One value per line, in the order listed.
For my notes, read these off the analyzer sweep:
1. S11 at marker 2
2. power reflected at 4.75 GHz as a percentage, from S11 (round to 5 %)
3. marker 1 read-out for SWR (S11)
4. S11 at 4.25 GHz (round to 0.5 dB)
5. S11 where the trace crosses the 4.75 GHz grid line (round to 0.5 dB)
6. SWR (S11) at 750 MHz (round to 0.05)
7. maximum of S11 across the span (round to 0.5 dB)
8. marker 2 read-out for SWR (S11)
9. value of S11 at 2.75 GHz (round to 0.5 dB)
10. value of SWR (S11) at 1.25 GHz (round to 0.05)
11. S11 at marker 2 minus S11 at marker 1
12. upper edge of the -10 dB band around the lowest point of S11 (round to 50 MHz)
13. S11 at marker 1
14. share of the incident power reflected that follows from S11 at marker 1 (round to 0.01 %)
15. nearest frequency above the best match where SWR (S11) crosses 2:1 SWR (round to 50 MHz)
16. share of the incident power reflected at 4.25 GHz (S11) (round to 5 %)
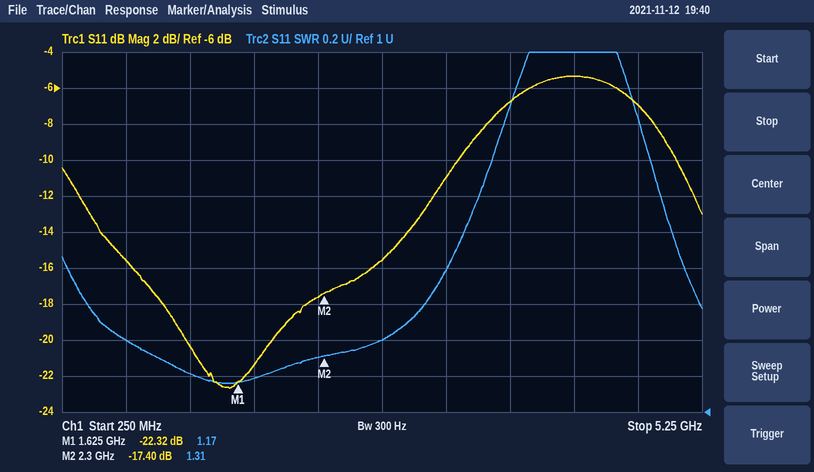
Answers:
-17.40 dB
20 %
1.17
-5.5 dB
-7.0 dB
1.40
-5.5 dB
1.31
-15.5 dB
1.20
4.92 dB
3.35 GHz
-22.32 dB
0.59 %
3.40 GHz
30 %
